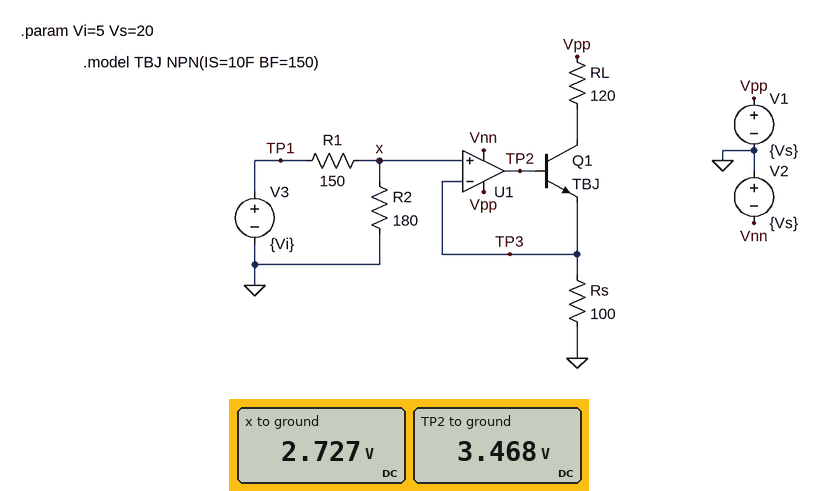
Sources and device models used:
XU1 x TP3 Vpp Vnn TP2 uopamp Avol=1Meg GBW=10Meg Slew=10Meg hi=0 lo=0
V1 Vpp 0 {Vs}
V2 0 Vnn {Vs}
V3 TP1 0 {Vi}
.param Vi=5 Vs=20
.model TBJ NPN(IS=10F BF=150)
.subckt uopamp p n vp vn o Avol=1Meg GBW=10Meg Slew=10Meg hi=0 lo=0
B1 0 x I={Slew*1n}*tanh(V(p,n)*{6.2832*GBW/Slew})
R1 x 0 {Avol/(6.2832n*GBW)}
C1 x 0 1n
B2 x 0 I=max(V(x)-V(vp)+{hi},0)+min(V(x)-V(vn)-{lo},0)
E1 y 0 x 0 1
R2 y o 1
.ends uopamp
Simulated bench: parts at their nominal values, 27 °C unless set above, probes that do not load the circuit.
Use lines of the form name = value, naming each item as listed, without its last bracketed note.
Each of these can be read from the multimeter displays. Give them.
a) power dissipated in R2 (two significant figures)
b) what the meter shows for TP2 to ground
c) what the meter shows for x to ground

power dissipated in R2 = 41 mW
what the meter shows for TP2 to ground = 3.468 V
what the meter shows for x to ground = 2.727 V
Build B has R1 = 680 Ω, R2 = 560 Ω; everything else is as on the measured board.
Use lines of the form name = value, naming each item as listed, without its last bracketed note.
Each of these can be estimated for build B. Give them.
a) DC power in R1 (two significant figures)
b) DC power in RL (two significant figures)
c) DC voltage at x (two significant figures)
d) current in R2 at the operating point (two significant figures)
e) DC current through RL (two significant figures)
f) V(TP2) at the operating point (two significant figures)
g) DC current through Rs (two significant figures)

DC power in R1 = 11 mW
DC power in RL = 60 mW
DC voltage at x = 2.3 V
current in R2 at the operating point = 4.0 mA
DC current through RL = 22 mA
V(TP2) at the operating point = 3.0 V
DC current through Rs = 23 mA
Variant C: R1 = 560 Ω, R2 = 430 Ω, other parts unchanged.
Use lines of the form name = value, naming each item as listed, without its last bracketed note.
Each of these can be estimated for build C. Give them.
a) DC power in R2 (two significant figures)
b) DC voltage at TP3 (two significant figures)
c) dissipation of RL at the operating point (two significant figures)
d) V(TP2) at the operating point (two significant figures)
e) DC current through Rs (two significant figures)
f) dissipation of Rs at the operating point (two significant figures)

DC power in R2 = 11 mW
DC voltage at TP3 = 2.2 V
dissipation of RL at the operating point = 56 mW
V(TP2) at the operating point = 2.9 V
DC current through Rs = 22 mA
dissipation of Rs at the operating point = 47 mW
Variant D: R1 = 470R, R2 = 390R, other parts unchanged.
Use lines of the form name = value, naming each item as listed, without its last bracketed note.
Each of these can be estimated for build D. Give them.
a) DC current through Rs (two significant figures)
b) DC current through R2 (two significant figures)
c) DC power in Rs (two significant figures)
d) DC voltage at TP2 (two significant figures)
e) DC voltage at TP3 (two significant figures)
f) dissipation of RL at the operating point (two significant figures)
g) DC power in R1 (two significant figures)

DC current through Rs = 23 mA
DC current through R2 = 5.8 mA
DC power in Rs = 51 mW
DC voltage at TP2 = 3.0 V
DC voltage at TP3 = 2.3 V
dissipation of RL at the operating point = 61 mW
DC power in R1 = 16 mW
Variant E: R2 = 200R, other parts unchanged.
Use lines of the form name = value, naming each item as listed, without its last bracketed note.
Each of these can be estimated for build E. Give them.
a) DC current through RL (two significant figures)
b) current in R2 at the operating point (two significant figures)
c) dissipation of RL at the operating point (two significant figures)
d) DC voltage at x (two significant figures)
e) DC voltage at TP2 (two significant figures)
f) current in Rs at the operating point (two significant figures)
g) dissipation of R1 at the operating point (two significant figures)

DC current through RL = 28 mA
current in R2 at the operating point = 14 mA
dissipation of RL at the operating point = 97 mW
DC voltage at x = 2.9 V
DC voltage at TP2 = 3.6 V
current in Rs at the operating point = 29 mA
dissipation of R1 at the operating point = 31 mW
